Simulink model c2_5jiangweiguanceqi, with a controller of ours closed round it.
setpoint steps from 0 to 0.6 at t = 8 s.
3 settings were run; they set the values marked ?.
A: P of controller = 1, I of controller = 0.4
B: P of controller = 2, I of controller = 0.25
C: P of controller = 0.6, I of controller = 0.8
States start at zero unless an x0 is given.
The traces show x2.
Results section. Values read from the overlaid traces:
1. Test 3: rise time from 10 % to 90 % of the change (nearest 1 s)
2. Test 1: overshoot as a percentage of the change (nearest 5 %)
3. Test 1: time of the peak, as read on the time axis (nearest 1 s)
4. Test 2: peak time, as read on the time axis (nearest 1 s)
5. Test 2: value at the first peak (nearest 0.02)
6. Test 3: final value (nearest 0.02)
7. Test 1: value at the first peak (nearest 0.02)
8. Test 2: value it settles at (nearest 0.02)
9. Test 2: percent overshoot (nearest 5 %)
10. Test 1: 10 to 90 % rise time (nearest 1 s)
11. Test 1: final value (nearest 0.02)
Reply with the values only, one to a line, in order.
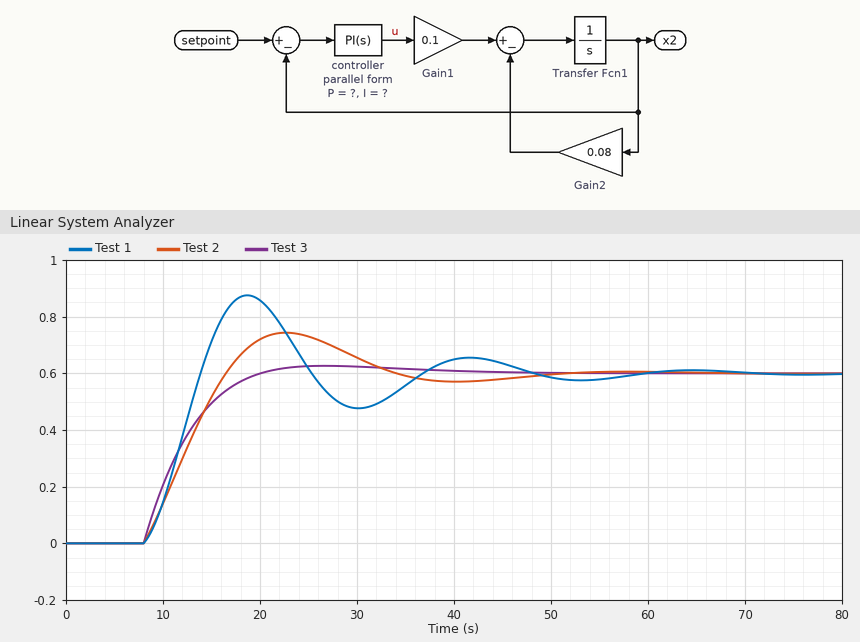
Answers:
8 s
45 %
19 s
23 s
0.74
0.60
0.88
0.60
25 %
4 s
0.60
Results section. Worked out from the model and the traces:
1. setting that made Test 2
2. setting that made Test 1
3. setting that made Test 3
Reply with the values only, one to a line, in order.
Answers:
A
C
B
